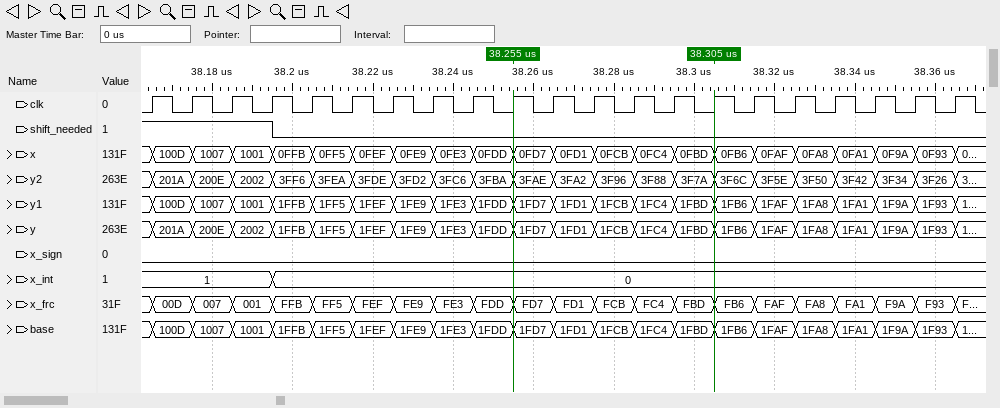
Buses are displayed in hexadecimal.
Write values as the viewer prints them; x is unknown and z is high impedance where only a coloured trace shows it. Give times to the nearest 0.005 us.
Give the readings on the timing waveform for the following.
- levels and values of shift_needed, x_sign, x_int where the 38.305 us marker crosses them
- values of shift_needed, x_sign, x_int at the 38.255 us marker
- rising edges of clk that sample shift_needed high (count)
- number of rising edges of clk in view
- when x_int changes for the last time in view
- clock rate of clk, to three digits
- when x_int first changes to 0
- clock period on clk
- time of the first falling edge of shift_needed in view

shift_needed=0, x_sign=0, x_int=0
shift_needed=0, x_sign=0, x_int=0
4
21
38.195 us
100 MHz
38.195 us
0.01 us
38.195 us
